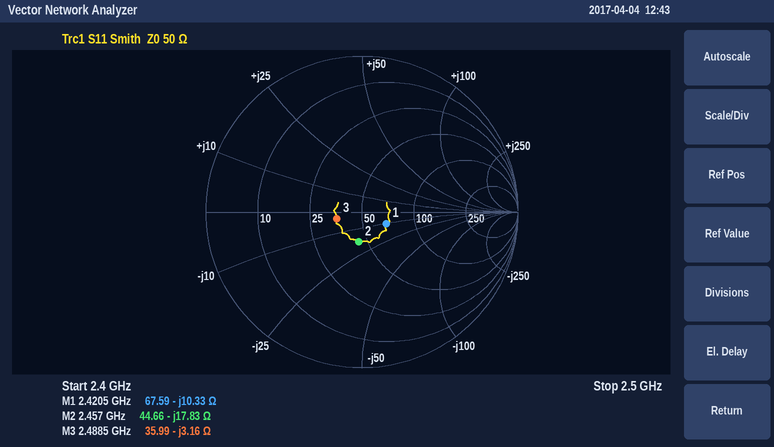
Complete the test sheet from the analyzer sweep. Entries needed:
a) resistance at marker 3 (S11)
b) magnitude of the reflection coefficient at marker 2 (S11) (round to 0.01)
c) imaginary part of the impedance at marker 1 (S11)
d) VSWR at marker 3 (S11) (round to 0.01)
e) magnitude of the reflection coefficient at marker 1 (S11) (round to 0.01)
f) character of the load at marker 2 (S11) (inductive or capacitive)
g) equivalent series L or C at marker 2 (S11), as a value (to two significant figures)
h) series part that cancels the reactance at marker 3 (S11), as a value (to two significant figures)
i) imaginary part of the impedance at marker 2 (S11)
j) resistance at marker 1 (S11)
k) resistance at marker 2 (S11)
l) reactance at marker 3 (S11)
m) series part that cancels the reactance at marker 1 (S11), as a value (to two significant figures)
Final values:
35.99 Ω
0.19
-10.33 Ω
1.40
0.17
capacitive
3.6 pF
200 pH
-17.83 Ω
67.59 Ω
44.66 Ω
-3.16 Ω
680 pH
